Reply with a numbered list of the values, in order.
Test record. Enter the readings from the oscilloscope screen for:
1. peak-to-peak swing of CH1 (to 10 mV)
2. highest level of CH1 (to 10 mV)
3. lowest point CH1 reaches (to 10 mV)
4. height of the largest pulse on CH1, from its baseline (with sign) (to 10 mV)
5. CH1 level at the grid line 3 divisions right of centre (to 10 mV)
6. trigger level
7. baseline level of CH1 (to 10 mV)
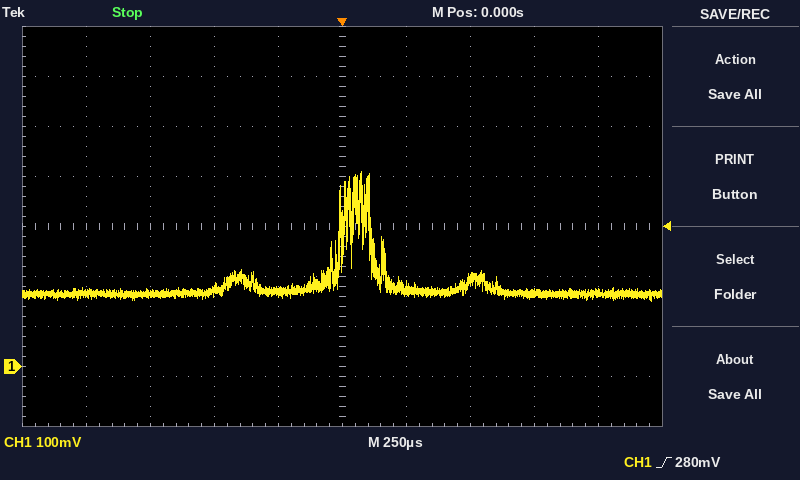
1. 260 mV
2. 390 mV
3. 130 mV
4. +240 mV
5. 150 mV
6. 280 mV
7. 150 mV
